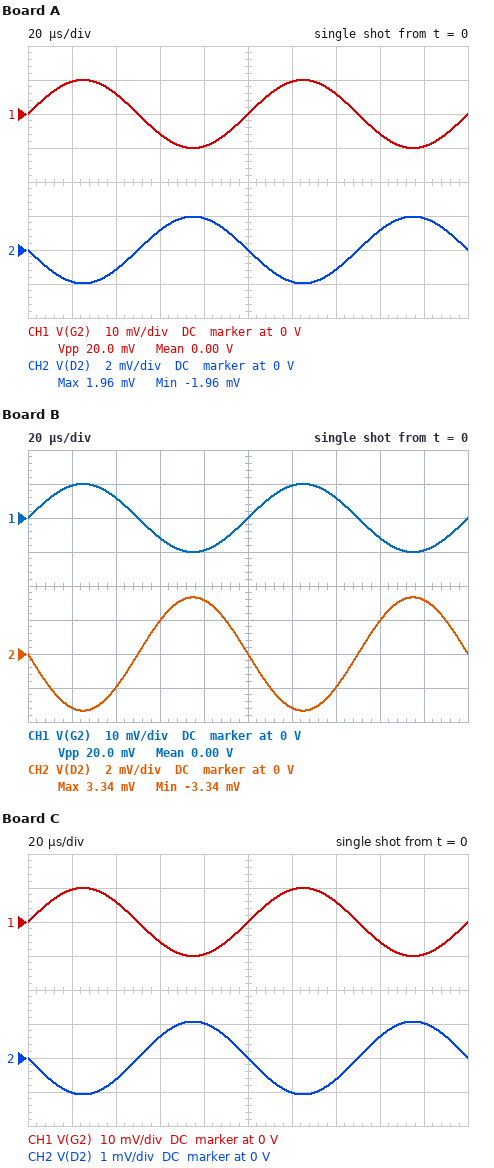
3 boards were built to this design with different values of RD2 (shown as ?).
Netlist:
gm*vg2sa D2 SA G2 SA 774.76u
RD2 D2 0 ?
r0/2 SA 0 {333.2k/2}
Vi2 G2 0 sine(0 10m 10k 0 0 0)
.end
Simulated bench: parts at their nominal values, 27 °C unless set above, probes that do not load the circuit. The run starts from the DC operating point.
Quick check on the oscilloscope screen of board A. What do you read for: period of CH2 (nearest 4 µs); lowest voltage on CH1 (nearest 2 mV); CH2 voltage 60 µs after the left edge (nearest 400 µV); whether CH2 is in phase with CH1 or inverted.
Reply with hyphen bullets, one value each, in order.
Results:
- 100 µs
- -10 mV
- 1.2 mV
- inverted
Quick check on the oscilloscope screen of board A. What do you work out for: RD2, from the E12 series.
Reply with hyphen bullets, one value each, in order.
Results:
- 33 kΩ
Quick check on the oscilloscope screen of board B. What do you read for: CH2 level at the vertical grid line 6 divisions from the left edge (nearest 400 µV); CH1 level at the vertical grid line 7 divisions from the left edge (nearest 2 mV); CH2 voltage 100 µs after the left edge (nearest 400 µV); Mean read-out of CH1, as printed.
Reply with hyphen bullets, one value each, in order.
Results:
- -3.2 mV
- 6 mV
- 0 V
- 0.00 V
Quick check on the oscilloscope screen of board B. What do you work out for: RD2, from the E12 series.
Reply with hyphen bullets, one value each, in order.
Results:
- 56 kΩ
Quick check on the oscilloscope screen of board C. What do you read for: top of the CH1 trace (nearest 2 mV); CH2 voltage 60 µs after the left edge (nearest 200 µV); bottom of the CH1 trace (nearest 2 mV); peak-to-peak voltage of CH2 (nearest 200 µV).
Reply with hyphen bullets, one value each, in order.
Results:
- 10 mV
- 600 µV
- -10 mV
- 2.2 mV
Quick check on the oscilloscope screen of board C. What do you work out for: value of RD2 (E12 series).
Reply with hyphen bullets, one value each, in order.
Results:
- 18 kΩ
